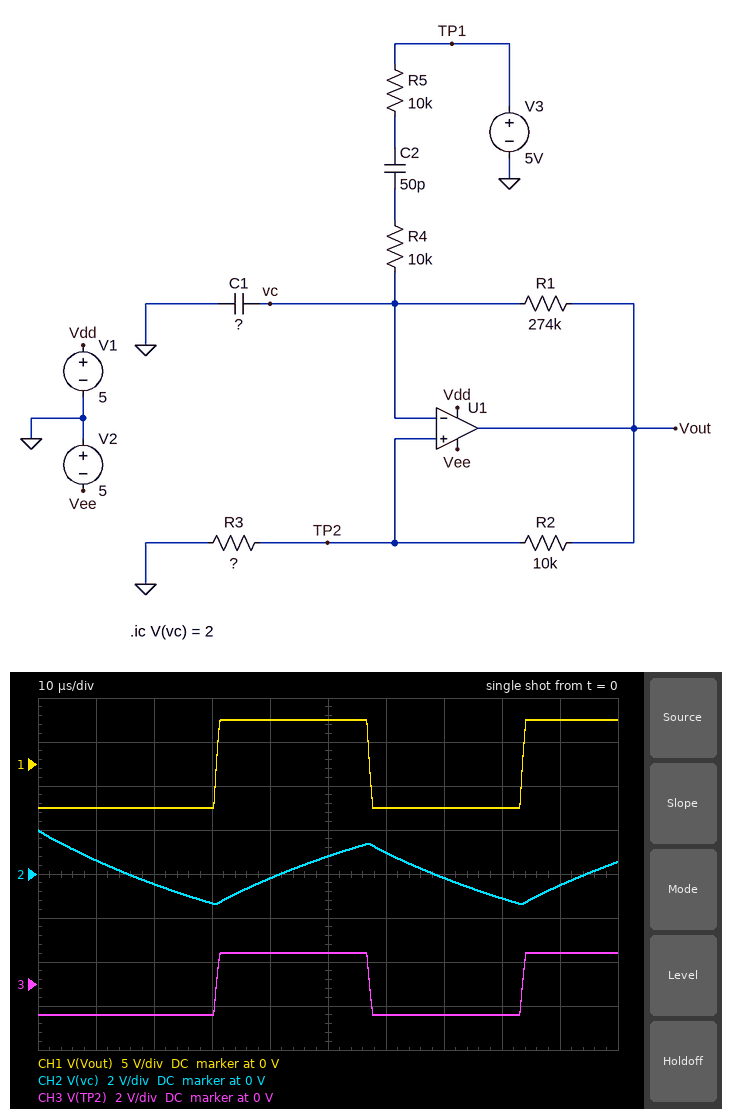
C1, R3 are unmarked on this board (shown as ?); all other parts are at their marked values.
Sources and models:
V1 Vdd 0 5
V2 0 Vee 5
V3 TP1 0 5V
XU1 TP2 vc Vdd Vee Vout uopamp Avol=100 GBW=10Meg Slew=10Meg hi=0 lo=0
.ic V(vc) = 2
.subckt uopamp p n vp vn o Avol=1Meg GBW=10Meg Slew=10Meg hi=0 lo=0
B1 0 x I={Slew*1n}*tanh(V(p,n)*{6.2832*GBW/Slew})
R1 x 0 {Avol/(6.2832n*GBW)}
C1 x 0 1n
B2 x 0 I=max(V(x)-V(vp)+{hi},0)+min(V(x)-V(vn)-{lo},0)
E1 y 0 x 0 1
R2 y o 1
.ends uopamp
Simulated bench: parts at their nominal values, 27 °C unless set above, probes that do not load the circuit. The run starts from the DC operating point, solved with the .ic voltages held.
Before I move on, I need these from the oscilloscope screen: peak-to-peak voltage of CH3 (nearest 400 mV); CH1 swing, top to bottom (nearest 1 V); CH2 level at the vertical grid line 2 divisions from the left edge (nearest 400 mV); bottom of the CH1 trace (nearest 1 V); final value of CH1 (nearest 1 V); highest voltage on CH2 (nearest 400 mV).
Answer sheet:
2.8 V
10 V
-400 mV
-5 V
5 V
2.0 V
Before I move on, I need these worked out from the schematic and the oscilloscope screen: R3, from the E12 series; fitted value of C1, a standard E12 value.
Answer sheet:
3.9 kΩ
120 pF
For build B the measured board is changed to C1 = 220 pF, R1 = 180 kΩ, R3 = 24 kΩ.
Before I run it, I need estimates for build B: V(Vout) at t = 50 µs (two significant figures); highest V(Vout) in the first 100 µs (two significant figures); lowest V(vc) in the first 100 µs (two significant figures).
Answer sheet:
-5.0 V
5.0 V
-3.5 V
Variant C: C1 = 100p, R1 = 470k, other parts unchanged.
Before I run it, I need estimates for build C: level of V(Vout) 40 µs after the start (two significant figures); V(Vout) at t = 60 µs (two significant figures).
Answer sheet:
-5.0 V
5.0 V
